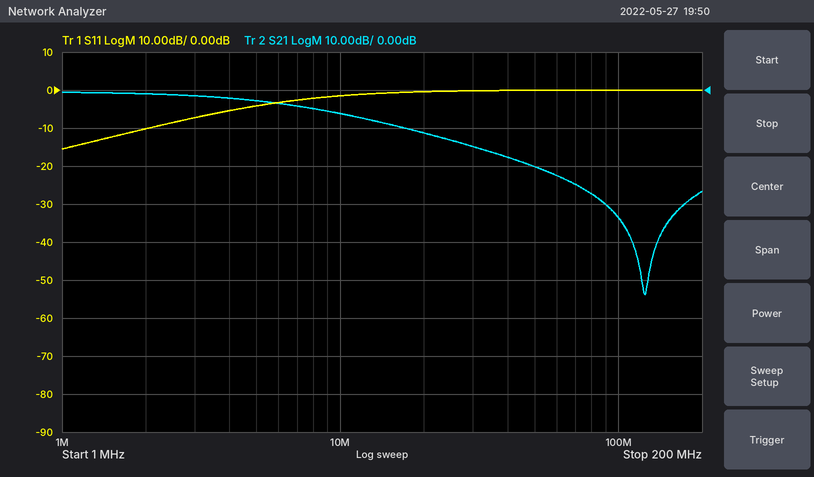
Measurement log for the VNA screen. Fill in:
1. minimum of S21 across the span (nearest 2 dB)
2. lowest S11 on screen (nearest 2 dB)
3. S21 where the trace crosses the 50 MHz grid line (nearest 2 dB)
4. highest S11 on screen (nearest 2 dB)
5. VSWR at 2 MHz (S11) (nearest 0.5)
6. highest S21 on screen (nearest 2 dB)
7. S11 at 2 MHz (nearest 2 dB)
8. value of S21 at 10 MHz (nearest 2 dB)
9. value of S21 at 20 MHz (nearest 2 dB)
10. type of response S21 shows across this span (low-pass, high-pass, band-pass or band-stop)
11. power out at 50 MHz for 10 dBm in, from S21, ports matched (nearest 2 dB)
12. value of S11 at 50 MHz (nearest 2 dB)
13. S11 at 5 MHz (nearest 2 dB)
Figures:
-54 dB
-16 dB
-20 dB
0 dB
2.0
0 dB
-10 dB
-6 dB
-12 dB
low-pass
-10 dBm
0 dB
-4 dB
